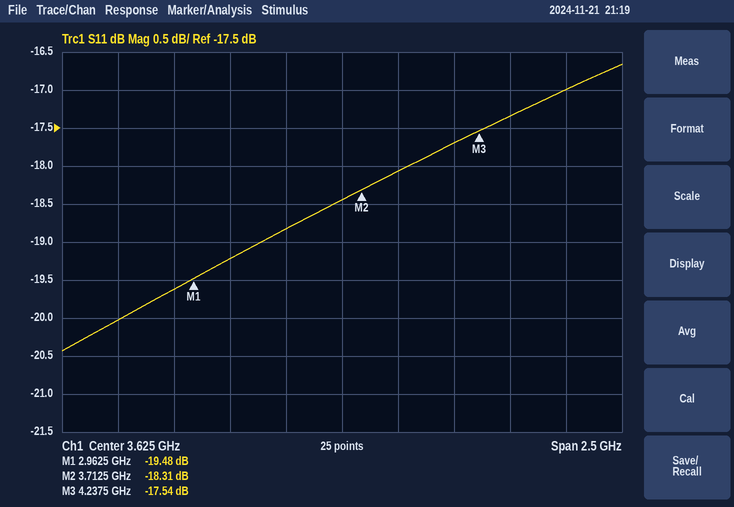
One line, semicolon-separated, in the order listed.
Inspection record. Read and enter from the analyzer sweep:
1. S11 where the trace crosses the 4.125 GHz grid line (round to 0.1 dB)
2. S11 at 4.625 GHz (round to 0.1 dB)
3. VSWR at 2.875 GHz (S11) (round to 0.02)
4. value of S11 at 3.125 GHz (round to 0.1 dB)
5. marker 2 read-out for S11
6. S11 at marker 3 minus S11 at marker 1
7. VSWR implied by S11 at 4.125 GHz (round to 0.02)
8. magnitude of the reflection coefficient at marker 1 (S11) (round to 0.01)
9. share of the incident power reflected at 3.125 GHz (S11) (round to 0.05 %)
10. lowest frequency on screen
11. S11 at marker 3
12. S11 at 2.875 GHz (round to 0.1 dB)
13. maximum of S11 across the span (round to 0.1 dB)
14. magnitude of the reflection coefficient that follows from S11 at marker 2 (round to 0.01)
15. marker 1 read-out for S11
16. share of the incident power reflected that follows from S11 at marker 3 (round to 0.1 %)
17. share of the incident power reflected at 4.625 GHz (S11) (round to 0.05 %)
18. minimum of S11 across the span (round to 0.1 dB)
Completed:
-17.7 dB; -17.0 dB; 1.24; -19.2 dB; -18.31 dB; 1.94 dB; 1.30; 0.11; 1.20 %; 2.375 GHz; -17.54 dB; -19.6 dB; -16.7 dB; 0.12; -19.48 dB; 1.8 %; 2.00 %; -20.4 dB
